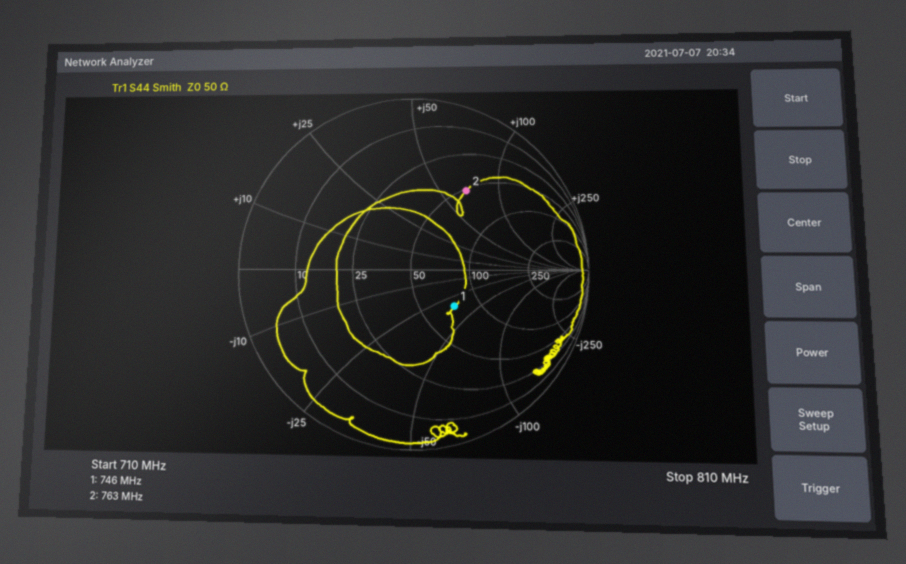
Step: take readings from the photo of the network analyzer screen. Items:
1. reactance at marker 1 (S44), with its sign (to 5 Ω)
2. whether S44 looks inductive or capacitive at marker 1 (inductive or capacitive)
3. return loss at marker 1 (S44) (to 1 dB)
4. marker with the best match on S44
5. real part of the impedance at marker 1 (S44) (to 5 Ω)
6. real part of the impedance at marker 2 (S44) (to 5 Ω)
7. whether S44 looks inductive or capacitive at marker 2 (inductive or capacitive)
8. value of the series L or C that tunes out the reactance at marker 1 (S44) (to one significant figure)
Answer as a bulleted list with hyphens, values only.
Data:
- -35 Ω
- capacitive
- 10 dB
- marker 1
- 75 Ω
- 50 Ω
- inductive
- 7 nH
